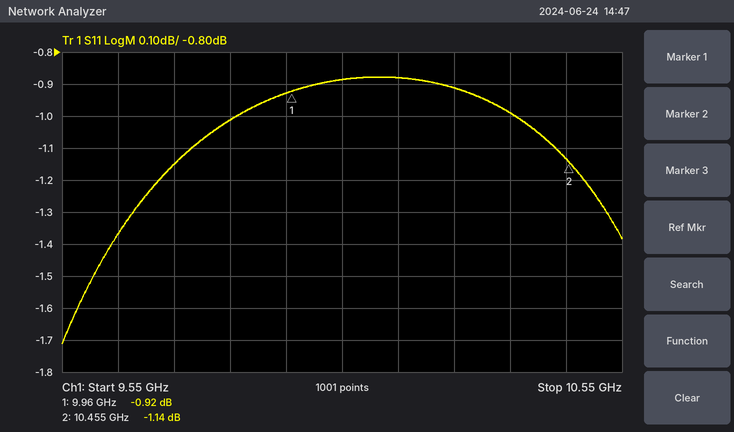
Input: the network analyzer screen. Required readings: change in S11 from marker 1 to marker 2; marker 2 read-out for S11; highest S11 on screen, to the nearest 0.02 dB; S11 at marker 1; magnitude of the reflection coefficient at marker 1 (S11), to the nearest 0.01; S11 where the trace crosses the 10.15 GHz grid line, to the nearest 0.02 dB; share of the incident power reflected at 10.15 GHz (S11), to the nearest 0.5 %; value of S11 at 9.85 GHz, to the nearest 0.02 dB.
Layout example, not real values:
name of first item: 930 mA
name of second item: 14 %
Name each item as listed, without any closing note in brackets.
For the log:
change in S11 from marker 1 to marker 2: -0.22 dB
marker 2 read-out for S11: -1.14 dB
highest S11 on screen, to the nearest 0.02 dB: -0.88 dB
S11 at marker 1: -0.92 dB
magnitude of the reflection coefficient at marker 1 (S11), to the nearest 0.01: 0.90
S11 where the trace crosses the 10.15 GHz grid line, to the nearest 0.02 dB: -0.88 dB
share of the incident power reflected at 10.15 GHz (S11), to the nearest 0.5 %: 81.5 %
value of S11 at 9.85 GHz, to the nearest 0.02 dB: -1.02 dB
